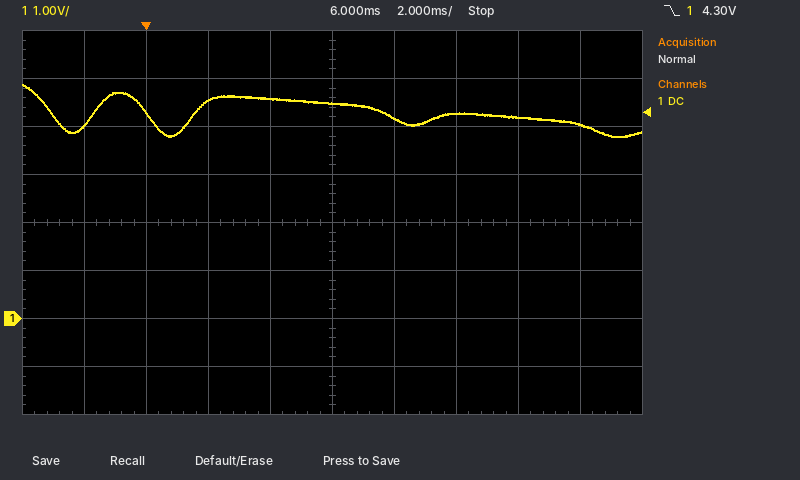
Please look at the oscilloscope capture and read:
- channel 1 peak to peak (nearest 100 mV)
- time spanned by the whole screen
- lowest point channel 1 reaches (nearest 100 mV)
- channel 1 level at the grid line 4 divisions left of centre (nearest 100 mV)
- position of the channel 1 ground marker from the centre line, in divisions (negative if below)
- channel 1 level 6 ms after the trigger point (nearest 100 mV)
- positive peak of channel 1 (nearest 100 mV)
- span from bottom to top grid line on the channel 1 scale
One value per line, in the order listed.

1.1 V
20 ms
3.8 V
4.0 V
-2.0 div
4.5 V
4.9 V
8 V
